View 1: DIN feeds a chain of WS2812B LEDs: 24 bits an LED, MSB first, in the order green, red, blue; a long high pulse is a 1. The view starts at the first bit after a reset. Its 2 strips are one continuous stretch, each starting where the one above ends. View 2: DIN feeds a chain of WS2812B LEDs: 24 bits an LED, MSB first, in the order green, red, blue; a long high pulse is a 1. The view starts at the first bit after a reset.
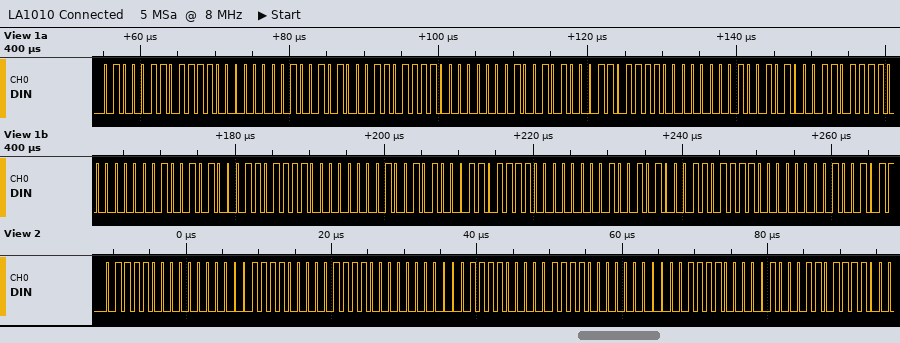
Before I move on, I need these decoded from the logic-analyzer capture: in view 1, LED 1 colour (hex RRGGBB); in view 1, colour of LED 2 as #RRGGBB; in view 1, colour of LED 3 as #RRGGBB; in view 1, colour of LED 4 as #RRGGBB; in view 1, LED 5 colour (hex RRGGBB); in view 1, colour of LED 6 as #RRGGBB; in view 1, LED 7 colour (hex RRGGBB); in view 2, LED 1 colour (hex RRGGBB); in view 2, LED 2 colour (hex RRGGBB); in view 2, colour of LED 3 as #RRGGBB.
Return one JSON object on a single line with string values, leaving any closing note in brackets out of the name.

{"in view 1, LED 1 colour": "#F04609", "in view 1, colour of LED 2 as #RRGGBB": "#F04609", "in view 1, colour of LED 3 as #RRGGBB": "#F04609", "in view 1, colour of LED 4 as #RRGGBB": "#F04609", "in view 1, LED 5 colour": "#F04609", "in view 1, colour of LED 6 as #RRGGBB": "#F04609", "in view 1, LED 7 colour": "#F04609", "in view 2, LED 1 colour": "#0078F0", "in view 2, LED 2 colour": "#0078F0", "in view 2, colour of LED 3 as #RRGGBB": "#0078F0"}
